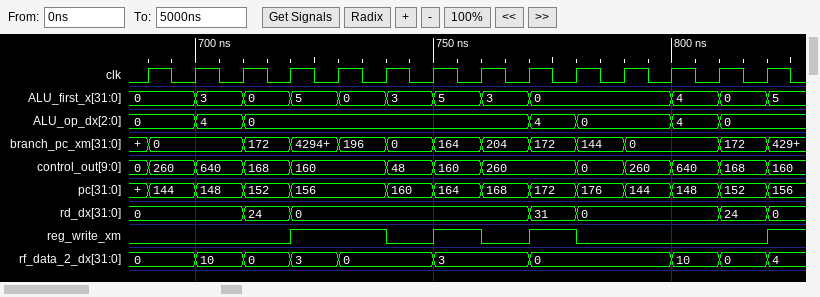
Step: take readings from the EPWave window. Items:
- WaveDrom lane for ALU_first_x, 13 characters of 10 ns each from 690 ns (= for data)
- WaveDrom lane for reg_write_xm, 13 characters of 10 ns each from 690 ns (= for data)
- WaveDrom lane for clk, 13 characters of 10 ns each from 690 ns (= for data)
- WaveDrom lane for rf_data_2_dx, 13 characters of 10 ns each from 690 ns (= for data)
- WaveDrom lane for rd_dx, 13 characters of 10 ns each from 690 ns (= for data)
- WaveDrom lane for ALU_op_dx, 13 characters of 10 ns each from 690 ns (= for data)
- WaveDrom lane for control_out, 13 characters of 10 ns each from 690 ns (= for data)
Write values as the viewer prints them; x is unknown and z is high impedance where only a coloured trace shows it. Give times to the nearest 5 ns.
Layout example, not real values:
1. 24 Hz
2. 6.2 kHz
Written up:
1. {name: 'ALU_first_x', wave: '=========..==', data: '0 3 0 5 0 3 5 3 0 4 0'}
2. {name: 'reg_write_xm', wave: '0..1.01010...'}
3. {name: 'clk', wave: 'p............'}
4. {name: 'rf_data_2_dx', wave: '=====.=.=..==', data: '0 10 0 3 0 3 0 10 0'}
5. {name: 'rd_dx', wave: '=.==....==..=', data: '0 24 0 31 0 24'}
6. {name: 'ALU_op_dx', wave: '===.....==.==', data: '0 4 0 4 0 4 0'}
7. {name: 'control_out', wave: '====.===.====', data: '260 640 168 160 48 160 260 0 260 640 168'}
